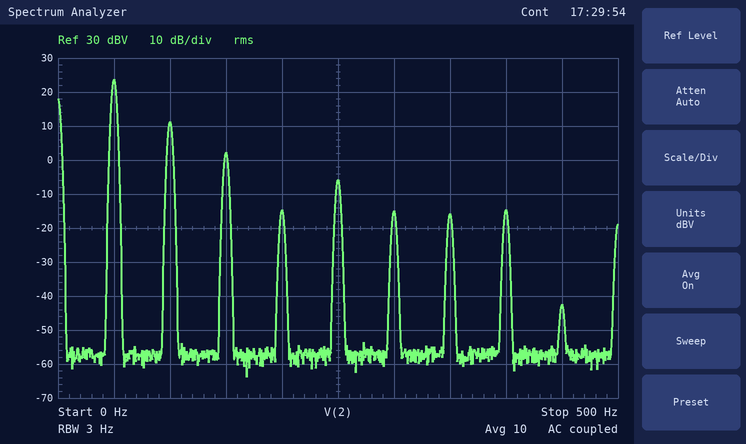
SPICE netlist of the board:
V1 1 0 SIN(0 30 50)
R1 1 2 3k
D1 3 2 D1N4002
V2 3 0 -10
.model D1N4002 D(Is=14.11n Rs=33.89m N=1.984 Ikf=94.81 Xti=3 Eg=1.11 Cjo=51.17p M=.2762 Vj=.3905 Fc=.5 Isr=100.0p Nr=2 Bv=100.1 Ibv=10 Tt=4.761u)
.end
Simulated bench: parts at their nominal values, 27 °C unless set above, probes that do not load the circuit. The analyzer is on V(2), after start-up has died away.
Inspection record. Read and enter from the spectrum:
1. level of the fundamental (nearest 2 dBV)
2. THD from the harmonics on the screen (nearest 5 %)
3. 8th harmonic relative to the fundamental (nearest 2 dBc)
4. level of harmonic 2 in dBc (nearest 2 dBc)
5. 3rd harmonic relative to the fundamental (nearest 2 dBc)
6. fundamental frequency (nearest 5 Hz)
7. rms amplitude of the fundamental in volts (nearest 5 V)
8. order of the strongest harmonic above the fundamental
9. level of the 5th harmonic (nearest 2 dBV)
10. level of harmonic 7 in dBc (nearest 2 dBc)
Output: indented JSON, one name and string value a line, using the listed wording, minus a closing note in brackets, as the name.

{
  "level of the fundamental": "24 dBV",
  "THD from the harmonics on the screen": "25 %",
  "8th harmonic relative to the fundamental": "-38 dBc",
  "level of harmonic 2 in dBc": "-12 dBc",
  "3rd harmonic relative to the fundamental": "-22 dBc",
  "fundamental frequency": "50 Hz",
  "rms amplitude of the fundamental in volts": "15 V",
  "order of the strongest harmonic above the fundamental": "2",
  "level of the 5th harmonic": "-6 dBV",
  "level of harmonic 7 in dBc": "-40 dBc"
}
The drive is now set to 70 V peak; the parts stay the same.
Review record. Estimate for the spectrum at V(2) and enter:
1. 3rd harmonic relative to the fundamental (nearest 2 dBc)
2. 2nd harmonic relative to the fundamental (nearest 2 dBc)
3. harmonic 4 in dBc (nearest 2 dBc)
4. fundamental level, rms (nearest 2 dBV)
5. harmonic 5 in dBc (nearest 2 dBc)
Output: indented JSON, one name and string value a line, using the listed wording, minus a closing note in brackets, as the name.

{
  "3rd harmonic relative to the fundamental": "-26 dBc",
  "2nd harmonic relative to the fundamental": "-10 dBc",
  "harmonic 4 in dBc": "-24 dBc",
  "fundamental level, rms": "30 dBV",
  "harmonic 5 in dBc": "-30 dBc"
}
